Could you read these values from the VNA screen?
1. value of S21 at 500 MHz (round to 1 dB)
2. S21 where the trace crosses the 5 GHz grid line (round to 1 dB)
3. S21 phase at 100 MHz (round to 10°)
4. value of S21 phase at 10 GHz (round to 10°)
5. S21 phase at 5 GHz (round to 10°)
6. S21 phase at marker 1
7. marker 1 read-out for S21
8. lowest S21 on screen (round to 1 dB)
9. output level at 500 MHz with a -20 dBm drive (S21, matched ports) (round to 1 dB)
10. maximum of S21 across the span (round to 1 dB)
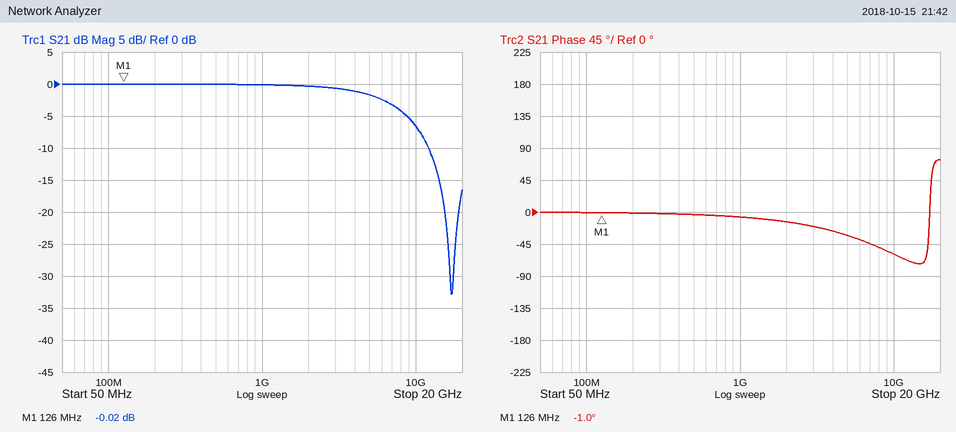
0 dB
-2 dB
0°
-60°
-30°
-1.0°
-0.02 dB
-33 dB
-20 dBm
0 dB
